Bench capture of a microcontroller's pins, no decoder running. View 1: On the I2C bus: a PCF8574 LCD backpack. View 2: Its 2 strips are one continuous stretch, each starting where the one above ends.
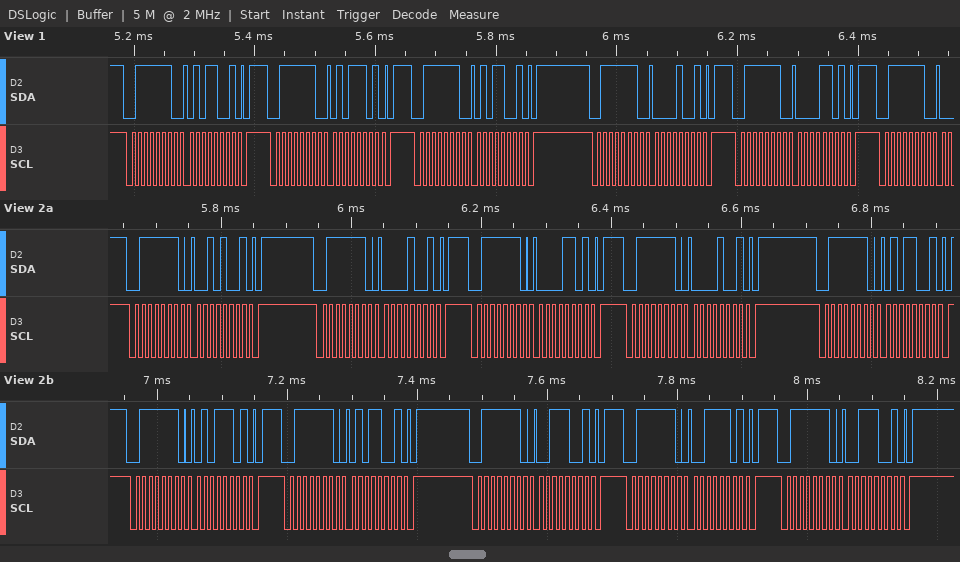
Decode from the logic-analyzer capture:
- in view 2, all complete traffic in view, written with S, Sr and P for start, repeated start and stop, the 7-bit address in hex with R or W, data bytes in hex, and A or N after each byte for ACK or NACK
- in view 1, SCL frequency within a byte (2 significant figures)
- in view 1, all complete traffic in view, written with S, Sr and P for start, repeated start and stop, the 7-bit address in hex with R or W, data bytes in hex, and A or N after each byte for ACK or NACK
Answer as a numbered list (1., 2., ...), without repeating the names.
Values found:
1. S 3FW A 29 A P S 3FW A 09 A P S 3FW A 0D A P S 3FW A 09 A P S 3FW A 59 A P S 3FW A 5D A P S 3FW A 59 A P S 3FW A 39 A P S 3FW A 3D A P S 3FW A 39 A P
2. 100 kHz
3. S 3FW A 59 A P S 3FW A 5D A P S 3FW A 59 A P S 3FW A 09 A P S 3FW A 0D A P S 3FW A
